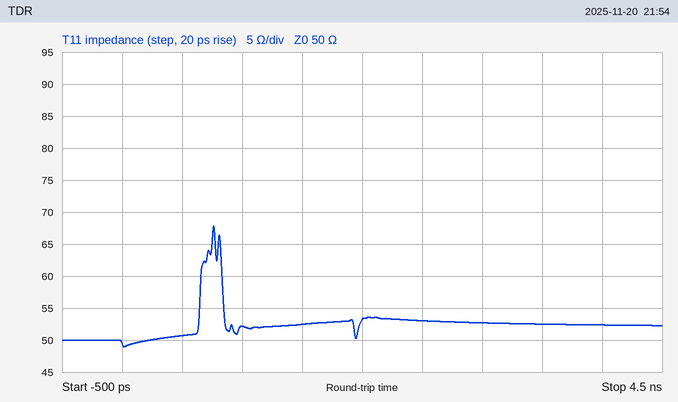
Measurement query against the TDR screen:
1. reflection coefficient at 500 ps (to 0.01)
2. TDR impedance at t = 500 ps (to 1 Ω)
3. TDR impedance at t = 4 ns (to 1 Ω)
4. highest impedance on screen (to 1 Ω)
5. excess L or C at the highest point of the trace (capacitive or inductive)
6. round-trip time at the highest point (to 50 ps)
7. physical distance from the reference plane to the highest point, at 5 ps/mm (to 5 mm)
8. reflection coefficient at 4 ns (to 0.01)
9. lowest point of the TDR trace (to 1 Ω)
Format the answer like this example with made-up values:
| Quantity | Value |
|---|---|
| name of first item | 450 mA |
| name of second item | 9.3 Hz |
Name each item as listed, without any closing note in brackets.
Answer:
| Quantity | Value |
|---|---|
| reflection coefficient at 500 ps | +0.01 |
| TDR impedance at t = 500 ps | 51 Ω |
| TDR impedance at t = 4 ns | 52 Ω |
| highest impedance on screen | 68 Ω |
| excess L or C at the highest point of the trace | inductive |
| round-trip time at the highest point | 750 ps |
| physical distance from the reference plane to the highest point, at 5 ps/mm | 75 mm |
| reflection coefficient at 4 ns | +0.02 |
| lowest point of the TDR trace | 49 Ω |
